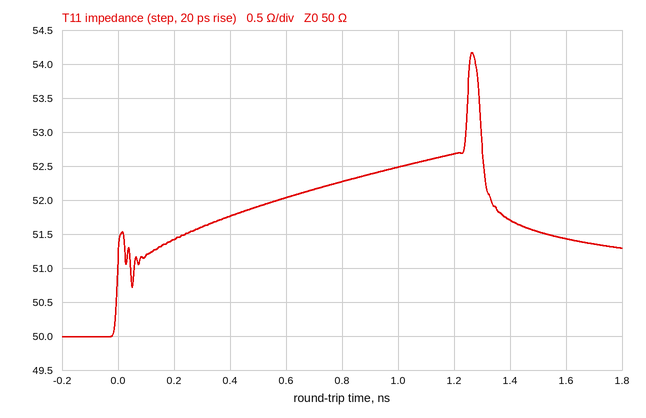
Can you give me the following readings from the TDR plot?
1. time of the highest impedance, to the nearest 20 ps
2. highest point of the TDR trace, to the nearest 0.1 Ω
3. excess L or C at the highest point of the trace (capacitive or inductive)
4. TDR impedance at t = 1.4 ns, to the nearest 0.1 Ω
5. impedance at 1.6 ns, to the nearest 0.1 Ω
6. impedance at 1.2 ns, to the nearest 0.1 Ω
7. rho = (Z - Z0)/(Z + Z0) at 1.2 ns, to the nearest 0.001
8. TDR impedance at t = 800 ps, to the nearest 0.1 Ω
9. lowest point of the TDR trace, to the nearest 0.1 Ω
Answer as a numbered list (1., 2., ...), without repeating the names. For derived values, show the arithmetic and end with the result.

1. 1.26 ns
2. 54.2 Ω
3. inductive
4. 51.7 Ω
5. 51.4 Ω
6. 52.7 Ω
7. (52.7 − 50)/(52.7 + 50) ≈ +0.026
8. 52.3 Ω
9. 50.0 Ω
